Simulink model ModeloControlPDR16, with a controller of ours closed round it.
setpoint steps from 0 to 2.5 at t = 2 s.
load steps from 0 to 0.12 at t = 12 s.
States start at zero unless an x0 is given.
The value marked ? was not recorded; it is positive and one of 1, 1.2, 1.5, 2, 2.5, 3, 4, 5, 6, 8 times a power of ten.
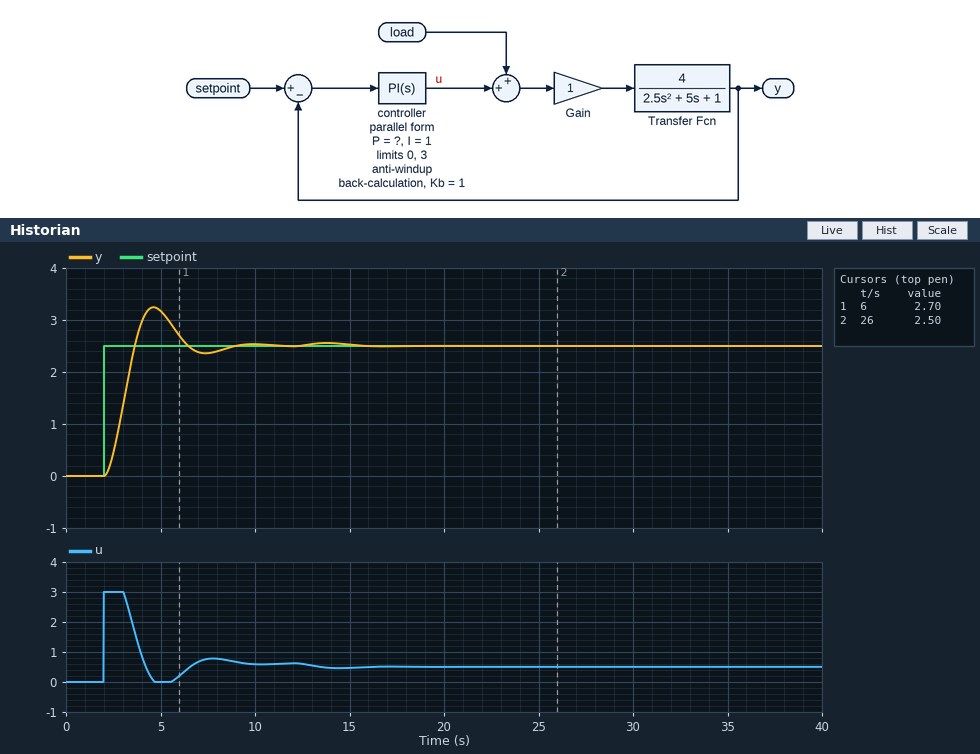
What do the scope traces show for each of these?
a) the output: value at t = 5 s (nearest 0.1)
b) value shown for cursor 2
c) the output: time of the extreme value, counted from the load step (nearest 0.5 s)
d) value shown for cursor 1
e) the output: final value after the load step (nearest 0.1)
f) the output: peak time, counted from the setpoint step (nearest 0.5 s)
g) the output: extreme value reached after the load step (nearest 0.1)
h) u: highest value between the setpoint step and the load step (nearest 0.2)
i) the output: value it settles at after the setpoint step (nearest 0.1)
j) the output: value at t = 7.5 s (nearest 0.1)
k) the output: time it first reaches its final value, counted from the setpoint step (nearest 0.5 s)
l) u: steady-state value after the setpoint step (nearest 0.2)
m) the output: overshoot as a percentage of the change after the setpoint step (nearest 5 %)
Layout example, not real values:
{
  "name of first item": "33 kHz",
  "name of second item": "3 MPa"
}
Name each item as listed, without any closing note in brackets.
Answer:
{
  "the output: value at t = 5 s": "3.2",
  "value shown for cursor 2": "2.50",
  "the output: time of the extreme value, counted from the load step": "2.0 s",
  "value shown for cursor 1": "2.70",
  "the output: final value after the load step": "2.5",
  "the output: peak time, counted from the setpoint step": "2.5 s",
  "the output: extreme value reached after the load step": "2.6",
  "u: highest value between the setpoint step and the load step": "3.0",
  "the output: value it settles at after the setpoint step": "2.5",
  "the output: value at t = 7.5 s": "2.4",
  "the output: time it first reaches its final value, counted from the setpoint step": "1.5 s",
  "u: steady-state value after the setpoint step": "0.6",
  "the output: overshoot as a percentage of the change after the setpoint step": "30 %"
}
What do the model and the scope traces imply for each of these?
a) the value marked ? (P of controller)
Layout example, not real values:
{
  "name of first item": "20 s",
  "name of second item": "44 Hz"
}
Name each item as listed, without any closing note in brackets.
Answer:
{
  "the value marked ?": "1.5"
}
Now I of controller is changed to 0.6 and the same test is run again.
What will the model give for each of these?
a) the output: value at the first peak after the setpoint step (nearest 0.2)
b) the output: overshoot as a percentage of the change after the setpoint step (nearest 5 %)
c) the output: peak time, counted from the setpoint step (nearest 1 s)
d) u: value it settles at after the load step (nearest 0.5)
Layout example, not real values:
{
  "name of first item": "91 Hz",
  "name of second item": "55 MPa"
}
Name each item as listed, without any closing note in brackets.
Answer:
{
  "the output: value at the first peak after the setpoint step": "3.0",
  "the output: overshoot as a percentage of the change after the setpoint step": "15 %",
  "the output: peak time, counted from the setpoint step": "3 s",
  "u: value it settles at after the load step": "0.5"
}
